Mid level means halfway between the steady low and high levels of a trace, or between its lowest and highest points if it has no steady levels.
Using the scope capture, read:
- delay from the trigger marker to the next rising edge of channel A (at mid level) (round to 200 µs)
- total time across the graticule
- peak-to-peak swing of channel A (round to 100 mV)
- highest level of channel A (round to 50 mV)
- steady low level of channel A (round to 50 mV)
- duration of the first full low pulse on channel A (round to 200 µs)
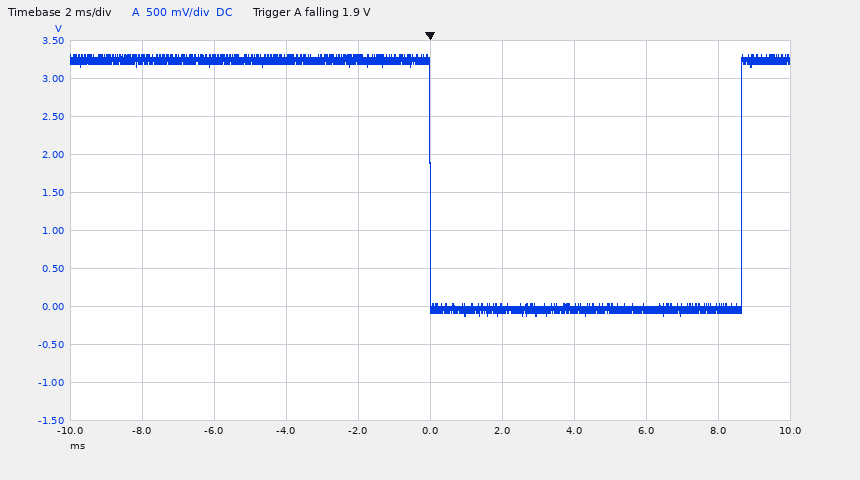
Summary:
8.6 ms
20 ms
3.40 V
3.30 V
-50 mV
8.6 ms
